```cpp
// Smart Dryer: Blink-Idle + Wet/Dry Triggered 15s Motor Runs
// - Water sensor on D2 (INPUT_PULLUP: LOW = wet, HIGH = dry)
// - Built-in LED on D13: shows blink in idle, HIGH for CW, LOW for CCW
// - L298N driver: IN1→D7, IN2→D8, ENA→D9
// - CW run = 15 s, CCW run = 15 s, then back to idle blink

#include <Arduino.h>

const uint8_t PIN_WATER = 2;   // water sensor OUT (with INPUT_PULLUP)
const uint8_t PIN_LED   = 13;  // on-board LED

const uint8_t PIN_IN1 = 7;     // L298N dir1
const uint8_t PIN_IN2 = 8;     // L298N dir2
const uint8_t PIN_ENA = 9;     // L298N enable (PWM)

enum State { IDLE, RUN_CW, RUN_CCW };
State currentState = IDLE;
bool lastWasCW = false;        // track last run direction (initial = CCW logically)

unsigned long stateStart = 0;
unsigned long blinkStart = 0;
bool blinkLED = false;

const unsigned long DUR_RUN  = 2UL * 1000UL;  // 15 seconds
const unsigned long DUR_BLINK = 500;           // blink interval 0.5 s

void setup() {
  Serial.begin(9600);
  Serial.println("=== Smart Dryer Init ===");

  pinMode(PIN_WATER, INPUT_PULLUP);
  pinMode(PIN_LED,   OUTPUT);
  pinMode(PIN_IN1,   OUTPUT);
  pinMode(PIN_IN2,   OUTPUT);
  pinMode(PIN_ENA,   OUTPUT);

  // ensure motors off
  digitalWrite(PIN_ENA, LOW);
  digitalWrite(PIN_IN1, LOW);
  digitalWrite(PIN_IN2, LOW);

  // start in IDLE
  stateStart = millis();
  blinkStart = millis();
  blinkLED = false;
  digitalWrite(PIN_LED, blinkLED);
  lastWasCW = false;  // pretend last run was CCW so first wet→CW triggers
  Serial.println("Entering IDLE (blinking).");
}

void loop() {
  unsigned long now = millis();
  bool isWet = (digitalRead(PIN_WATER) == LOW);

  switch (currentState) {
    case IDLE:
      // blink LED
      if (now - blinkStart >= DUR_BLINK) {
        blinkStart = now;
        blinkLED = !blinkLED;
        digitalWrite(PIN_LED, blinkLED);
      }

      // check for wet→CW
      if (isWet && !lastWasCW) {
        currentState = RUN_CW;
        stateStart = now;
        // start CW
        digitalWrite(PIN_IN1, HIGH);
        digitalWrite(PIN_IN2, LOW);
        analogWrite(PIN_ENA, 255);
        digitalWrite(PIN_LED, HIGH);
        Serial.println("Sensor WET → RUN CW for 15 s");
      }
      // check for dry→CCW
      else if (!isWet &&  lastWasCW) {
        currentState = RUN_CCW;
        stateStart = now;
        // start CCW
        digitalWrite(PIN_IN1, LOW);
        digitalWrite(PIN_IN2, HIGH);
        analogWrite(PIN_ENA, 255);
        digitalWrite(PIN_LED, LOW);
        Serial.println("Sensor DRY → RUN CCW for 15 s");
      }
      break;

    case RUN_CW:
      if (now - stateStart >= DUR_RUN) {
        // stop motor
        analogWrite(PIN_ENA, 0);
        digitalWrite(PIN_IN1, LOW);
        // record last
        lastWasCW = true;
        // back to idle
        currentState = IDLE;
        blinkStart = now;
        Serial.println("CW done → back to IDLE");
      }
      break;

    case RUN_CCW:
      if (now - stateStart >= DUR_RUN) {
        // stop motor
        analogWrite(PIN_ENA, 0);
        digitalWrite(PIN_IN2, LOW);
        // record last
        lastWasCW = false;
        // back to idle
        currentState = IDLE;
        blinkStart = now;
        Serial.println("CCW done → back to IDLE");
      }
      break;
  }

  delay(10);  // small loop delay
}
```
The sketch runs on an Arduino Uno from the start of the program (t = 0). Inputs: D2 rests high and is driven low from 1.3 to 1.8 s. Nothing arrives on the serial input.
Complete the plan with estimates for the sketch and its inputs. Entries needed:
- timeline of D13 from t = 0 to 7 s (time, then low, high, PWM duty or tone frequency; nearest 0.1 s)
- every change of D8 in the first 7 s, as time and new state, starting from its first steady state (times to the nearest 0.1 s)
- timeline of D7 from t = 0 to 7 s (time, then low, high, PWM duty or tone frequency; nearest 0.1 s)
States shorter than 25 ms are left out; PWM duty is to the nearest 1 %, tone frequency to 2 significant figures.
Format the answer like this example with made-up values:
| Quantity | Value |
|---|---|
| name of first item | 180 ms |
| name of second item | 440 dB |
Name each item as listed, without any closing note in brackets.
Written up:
| Quantity | Value |
|---|---|
| timeline of D13 from t = 0 to 7 s | 0 s low; 0.5 s high; 1 s low; 1.3 s high; 3.3 s low; 5.8 s high; 6.3 s low; 6.8 s high |
| every change of D8 in the first 7 s, as time and new state, starting from its first steady state | 0 s low; 3.3 s high; 5.3 s low |
| timeline of D7 from t = 0 to 7 s | 0 s low; 1.3 s high; 3.3 s low |
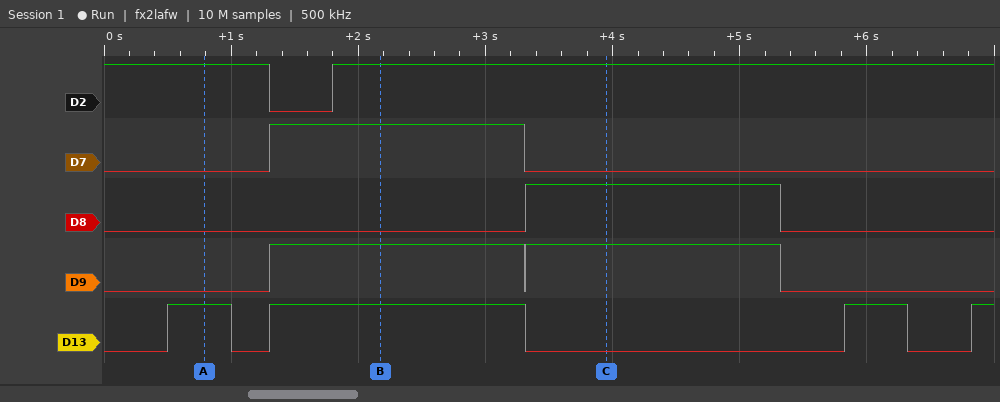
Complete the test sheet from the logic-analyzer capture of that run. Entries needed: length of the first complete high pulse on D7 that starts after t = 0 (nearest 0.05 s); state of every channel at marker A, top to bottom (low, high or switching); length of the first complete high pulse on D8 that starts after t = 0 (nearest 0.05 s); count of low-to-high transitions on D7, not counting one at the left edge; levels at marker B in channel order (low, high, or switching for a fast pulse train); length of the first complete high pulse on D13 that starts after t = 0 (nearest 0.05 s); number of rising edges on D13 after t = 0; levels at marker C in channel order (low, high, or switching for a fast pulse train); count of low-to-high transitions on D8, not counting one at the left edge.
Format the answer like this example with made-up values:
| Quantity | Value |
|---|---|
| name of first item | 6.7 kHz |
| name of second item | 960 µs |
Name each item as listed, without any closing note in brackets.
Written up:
| Quantity | Value |
|---|---|
| length of the first complete high pulse on D7 that starts after t = 0 | 2.00 s |
| state of every channel at marker A, top to bottom | D2 high, D7 low, D8 low, D9 low, D13 high |
| length of the first complete high pulse on D8 that starts after t = 0 | 2.00 s |
| count of low-to-high transitions on D7, not counting one at the left edge | 1 |
| levels at marker B in channel order | D2 high, D7 high, D8 low, D9 high, D13 high |
| length of the first complete high pulse on D13 that starts after t = 0 | 0.50 s |
| number of rising edges on D13 after t = 0 | 4 |
| levels at marker C in channel order | D2 high, D7 low, D8 high, D9 high, D13 low |
| count of low-to-high transitions on D8, not counting one at the left edge | 1 |
